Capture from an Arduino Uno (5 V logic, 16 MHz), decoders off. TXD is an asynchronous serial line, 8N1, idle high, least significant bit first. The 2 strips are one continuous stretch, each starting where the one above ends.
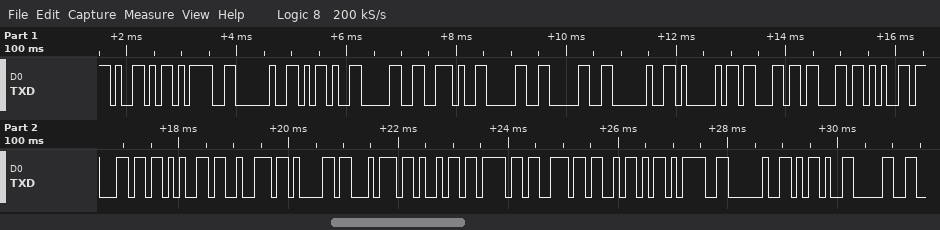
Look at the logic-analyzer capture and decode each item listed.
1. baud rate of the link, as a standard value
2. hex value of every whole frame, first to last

9600 baud
59 3D 20 2D 30 2E 30 30 20 41 63 63 65 6C 65 72 61 74 69 6F 6E 5A 3D 20 2D 30
